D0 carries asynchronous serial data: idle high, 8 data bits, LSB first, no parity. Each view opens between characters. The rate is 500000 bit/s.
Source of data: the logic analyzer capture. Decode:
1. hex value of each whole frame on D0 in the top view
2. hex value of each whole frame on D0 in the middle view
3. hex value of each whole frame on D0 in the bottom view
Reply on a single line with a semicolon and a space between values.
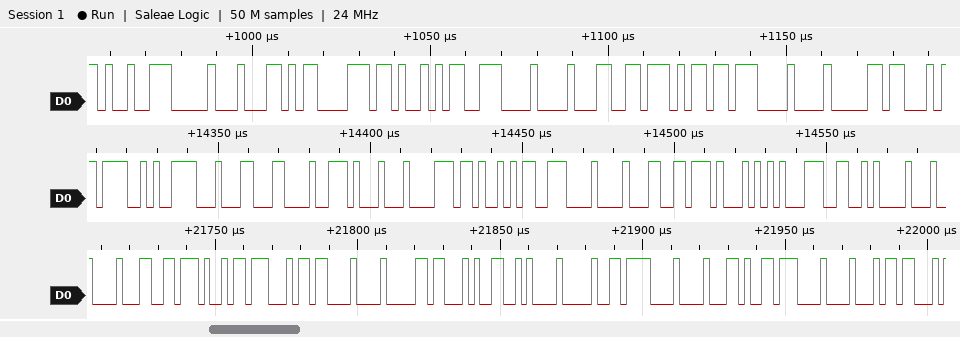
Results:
C9, 10, AC, B8, A9, 0E, 88, 76, DB, 08, B0; 4F, 1E, 8C, C8, 11, B8, A9, 0E, 88, 76, 54, 9C, 0A; 88, 76, DA, B4, 08, B0, 94, 0A, 90, 0F, 88, D9, 08, B4
